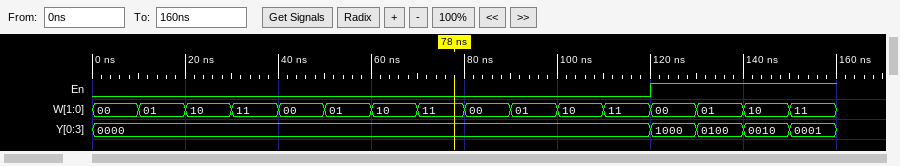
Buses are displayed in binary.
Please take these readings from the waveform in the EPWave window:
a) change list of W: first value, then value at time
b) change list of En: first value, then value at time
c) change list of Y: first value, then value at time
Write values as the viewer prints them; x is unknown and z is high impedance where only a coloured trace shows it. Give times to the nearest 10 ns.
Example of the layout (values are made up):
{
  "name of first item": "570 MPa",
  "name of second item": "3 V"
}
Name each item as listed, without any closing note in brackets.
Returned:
{
  "change list of W: first value, then value at time": "00, 01 at 10 ns, 10 at 20 ns, 11 at 30 ns, 00 at 40 ns, 01 at 50 ns, 10 at 60 ns, 11 at 70 ns, 00 at 80 ns, 01 at 90 ns, 10 at 100 ns, 11 at 110 ns, 00 at 120 ns, 01 at 130 ns, 10 at 140 ns, 11 at 150 ns",
  "change list of En: first value, then value at time": "0, 1 at 120 ns",
  "change list of Y: first value, then value at time": "0000, 1000 at 120 ns, 0100 at 130 ns, 0010 at 140 ns, 0001 at 150 ns"
}
